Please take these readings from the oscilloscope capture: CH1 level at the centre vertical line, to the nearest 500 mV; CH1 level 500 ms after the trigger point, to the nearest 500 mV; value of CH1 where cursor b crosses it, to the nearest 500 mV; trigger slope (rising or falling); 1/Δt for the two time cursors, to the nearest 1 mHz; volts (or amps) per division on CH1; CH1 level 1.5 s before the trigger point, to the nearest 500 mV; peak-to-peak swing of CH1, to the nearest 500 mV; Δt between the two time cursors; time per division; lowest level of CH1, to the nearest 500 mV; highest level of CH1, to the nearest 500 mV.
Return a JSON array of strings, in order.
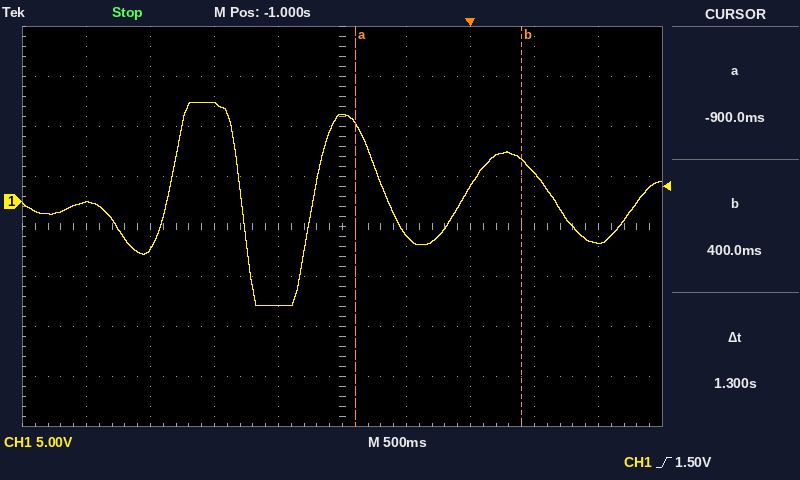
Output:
["8.5 V", "3.0 V", "4.0 V", "rising", "769 mHz", "5 V", "-10.5 V", "20.5 V", "1.3 s", "500 ms", "-10.5 V", "10.0 V"]
